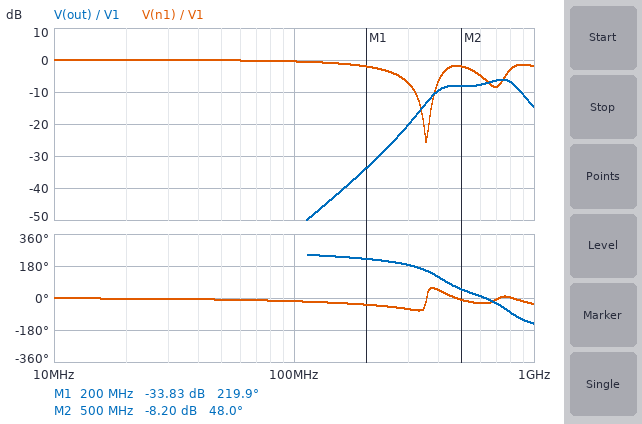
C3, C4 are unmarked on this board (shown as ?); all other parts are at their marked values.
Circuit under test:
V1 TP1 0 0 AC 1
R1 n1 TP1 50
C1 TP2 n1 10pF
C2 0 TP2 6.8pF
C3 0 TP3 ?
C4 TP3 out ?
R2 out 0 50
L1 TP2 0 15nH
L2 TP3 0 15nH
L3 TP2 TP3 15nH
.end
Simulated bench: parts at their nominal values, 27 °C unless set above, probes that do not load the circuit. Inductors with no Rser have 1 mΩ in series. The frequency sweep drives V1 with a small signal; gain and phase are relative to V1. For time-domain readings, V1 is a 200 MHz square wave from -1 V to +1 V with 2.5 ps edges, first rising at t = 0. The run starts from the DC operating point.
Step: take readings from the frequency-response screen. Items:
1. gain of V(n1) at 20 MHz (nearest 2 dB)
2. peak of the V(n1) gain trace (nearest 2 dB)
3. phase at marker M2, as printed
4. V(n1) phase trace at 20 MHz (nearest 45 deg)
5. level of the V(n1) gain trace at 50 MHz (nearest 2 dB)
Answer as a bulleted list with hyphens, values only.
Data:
- 0 dB
- 0 dB
- 48.0 deg
- 0 deg
- 0 dB
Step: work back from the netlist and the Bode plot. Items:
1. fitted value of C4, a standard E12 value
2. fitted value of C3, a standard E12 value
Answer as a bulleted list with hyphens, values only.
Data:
- 3.3 pF
- 5.6 pF
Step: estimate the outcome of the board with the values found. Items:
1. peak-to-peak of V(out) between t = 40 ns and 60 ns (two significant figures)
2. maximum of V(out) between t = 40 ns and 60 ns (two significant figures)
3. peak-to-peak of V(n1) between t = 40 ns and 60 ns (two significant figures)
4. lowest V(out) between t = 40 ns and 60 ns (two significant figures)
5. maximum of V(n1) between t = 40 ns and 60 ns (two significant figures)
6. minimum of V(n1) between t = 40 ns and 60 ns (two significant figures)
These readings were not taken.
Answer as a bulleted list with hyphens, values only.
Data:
- 470 mV
- 230 mV
- 2.5 V
- -230 mV
- 1.2 V
- -1.2 V
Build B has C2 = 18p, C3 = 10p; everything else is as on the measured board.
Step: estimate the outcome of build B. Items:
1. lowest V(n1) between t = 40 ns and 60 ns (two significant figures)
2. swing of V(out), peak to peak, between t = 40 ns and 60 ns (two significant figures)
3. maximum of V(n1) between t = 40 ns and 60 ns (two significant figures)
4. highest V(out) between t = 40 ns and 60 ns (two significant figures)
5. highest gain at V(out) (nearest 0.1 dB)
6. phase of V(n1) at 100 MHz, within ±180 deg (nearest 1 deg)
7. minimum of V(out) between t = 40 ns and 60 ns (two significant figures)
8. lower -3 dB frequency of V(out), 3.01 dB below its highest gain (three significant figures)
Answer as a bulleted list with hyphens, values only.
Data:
- -1.1 V
- 400 mV
- 1.1 V
- 200 mV
- -6.2 dB
- -18 deg
- -200 mV
- 523 MHz
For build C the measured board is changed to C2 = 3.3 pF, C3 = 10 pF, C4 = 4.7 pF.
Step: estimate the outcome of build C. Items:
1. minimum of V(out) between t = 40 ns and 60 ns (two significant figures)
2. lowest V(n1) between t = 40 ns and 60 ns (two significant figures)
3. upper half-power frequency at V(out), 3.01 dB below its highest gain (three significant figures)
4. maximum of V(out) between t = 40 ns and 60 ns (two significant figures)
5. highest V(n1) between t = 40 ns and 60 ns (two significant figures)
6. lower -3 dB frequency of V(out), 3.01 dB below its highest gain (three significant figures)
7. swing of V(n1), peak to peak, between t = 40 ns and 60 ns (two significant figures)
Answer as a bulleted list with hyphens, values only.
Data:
- -180 mV
- -1.1 V
- 547 MHz
- 180 mV
- 1.1 V
- 355 MHz
- 2.3 V
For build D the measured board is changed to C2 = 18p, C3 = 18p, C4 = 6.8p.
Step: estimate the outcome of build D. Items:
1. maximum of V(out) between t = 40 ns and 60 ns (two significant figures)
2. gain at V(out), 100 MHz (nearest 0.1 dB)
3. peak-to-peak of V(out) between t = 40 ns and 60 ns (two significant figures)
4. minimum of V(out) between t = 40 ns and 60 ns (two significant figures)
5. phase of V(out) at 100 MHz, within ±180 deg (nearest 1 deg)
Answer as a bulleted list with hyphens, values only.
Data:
- 140 mV
- -46.2 dB
- 280 mV
- -140 mV
- -121 deg
